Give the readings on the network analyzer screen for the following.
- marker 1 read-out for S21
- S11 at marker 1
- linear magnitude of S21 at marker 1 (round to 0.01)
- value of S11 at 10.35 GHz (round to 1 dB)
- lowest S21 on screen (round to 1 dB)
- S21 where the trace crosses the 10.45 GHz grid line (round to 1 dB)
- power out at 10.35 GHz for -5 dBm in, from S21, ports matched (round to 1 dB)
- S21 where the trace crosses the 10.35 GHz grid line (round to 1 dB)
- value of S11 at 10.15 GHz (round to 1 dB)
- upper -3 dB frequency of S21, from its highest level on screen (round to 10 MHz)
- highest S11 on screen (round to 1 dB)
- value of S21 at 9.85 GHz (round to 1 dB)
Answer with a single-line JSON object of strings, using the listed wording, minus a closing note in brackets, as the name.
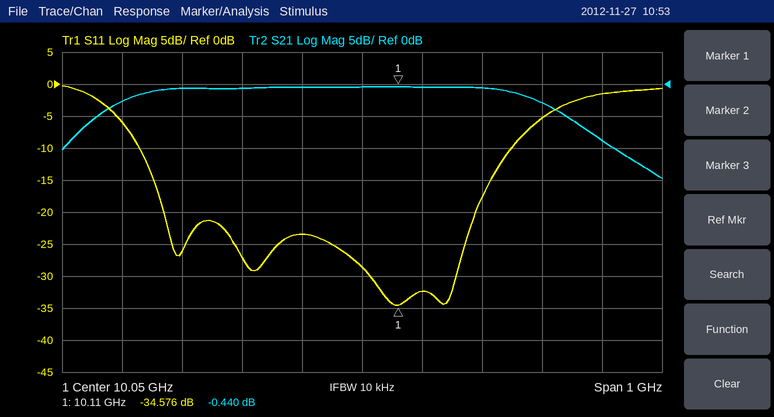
{"marker 1 read-out for S21": "-0.440 dB", "S11 at marker 1": "-34.576 dB", "linear magnitude of S21 at marker 1": "0.95", "value of S11 at 10.35 GHz": "-5 dB", "lowest S21 on screen": "-15 dB", "S21 where the trace crosses the 10.45 GHz grid line": "-9 dB", "power out at 10.35 GHz for -5 dBm in, from S21, ports matched": "-8 dBm", "S21 where the trace crosses the 10.35 GHz grid line": "-3 dB", "value of S11 at 10.15 GHz": "-32 dB", "upper -3 dB frequency of S21, from its highest level on screen": "10.36 GHz", "highest S11 on screen": "0 dB", "value of S21 at 9.85 GHz": "-1 dB"}
